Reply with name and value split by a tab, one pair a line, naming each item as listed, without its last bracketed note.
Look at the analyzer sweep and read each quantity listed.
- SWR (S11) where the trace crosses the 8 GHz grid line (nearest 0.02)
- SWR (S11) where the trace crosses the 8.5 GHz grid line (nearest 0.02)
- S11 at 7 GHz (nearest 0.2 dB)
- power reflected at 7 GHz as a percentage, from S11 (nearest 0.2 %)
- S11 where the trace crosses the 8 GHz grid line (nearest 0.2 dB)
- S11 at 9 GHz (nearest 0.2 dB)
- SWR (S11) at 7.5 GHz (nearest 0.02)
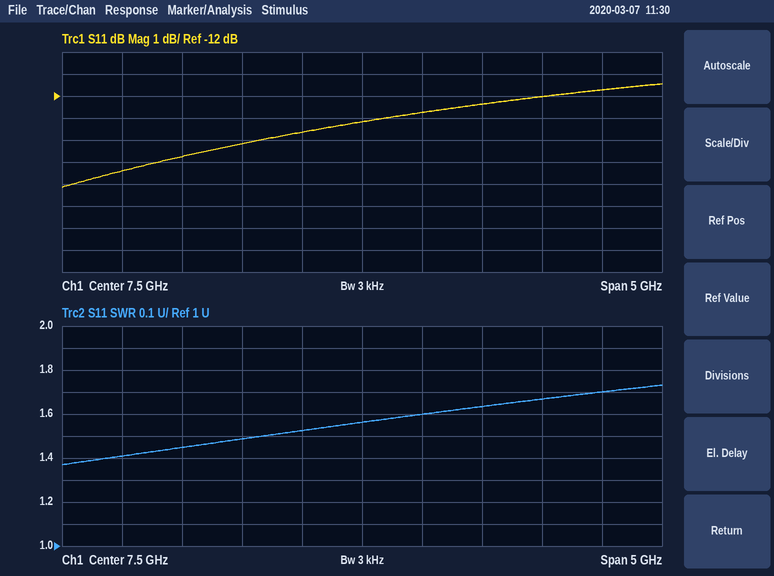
SWR (S11) where the trace crosses the 8 GHz grid line	1.60
SWR (S11) where the trace crosses the 8.5 GHz grid line	1.64
S11 at 7 GHz	-13.6 dB
power reflected at 7 GHz as a percentage, from S11	4.4 %
S11 where the trace crosses the 8 GHz grid line	-12.8 dB
S11 at 9 GHz	-12.0 dB
SWR (S11) at 7.5 GHz	1.56
